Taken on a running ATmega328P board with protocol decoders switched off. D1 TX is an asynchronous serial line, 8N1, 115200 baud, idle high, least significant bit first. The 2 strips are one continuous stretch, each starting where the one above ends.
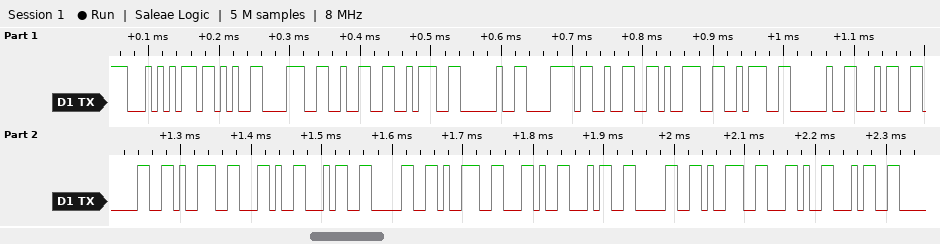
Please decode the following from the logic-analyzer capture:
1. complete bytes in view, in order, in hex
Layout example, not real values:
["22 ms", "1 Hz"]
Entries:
["0x54 0x2B 0x38 0x32 0x3A 0x20 0x78 0x32 0x39 0x3A 0x20 0x34 0x30 0x39 0x2C 0x34 0x30 0x39 0x2C 0x34 0x30 0x39 0x2C 0x34"]
